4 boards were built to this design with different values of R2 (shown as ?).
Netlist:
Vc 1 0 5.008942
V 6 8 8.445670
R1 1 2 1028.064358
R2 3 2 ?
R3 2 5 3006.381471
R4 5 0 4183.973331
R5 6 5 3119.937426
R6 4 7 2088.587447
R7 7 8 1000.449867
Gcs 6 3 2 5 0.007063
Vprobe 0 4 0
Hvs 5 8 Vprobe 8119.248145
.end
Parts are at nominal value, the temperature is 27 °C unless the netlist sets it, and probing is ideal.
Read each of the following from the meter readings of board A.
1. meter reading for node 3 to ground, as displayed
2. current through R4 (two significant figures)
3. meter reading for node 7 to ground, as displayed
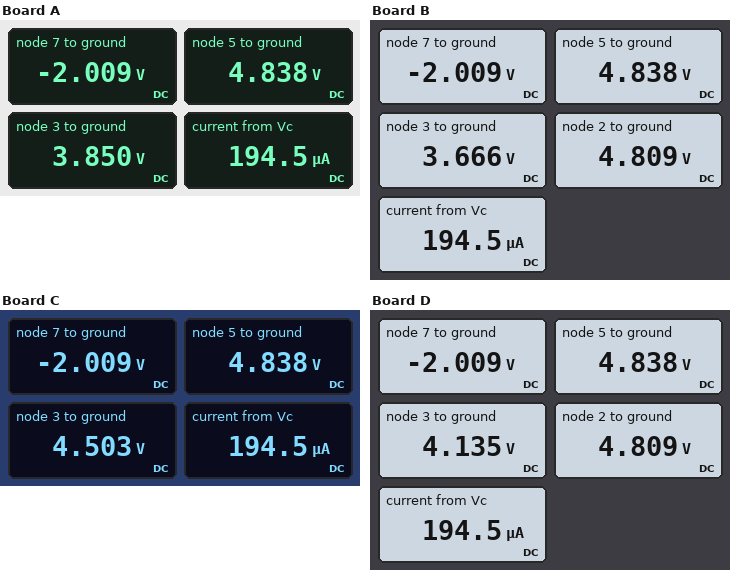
3.850 V
1.2 mA
-2.009 V
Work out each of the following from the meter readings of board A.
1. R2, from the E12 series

4.7 kΩ
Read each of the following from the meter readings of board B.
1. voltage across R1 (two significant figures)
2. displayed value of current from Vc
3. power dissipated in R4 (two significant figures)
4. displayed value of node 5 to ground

200 mV
194.5 µA
5.6 mW
4.838 V
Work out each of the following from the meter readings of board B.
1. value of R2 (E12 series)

5.6 kΩ
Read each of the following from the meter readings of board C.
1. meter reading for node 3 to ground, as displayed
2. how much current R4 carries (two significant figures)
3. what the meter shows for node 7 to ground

4.503 V
1.2 mA
-2.009 V
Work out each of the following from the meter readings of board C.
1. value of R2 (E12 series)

1.5 kΩ
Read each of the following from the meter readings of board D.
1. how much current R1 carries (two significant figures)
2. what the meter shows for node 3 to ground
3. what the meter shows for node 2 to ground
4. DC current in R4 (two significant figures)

190 µA
4.135 V
4.809 V
1.2 mA
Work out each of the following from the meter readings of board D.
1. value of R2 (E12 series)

3.3 kΩ
